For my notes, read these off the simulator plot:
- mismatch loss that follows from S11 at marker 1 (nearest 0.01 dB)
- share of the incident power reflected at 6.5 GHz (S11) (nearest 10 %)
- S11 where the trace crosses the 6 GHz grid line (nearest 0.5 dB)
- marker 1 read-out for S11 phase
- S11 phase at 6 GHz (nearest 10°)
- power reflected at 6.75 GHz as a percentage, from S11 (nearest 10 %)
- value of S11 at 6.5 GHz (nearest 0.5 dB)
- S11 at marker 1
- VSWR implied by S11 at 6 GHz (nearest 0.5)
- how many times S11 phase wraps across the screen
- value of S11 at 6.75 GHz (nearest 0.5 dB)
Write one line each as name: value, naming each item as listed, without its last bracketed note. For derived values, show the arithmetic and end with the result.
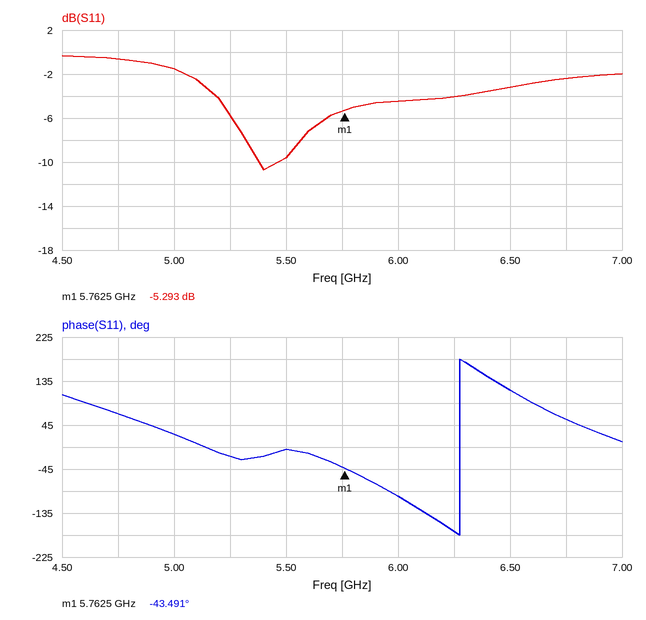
mismatch loss that follows from S11 at marker 1: −10 log10(1 − 10^(-5.293/10)) ≈ 1.52 dB
share of the incident power reflected at 6.5 GHz (S11): 10^(-3/10) ≈ 50 %
S11 where the trace crosses the 6 GHz grid line: -4.5 dB
marker 1 read-out for S11 phase: -43.491°
S11 phase at 6 GHz: -100°
power reflected at 6.75 GHz as a percentage, from S11: 10^(-2.5/10) ≈ 56.2 %, so 60 % to the nearest 10 %
value of S11 at 6.5 GHz: -3.0 dB
S11 at marker 1: -5.293 dB
VSWR implied by S11 at 6 GHz: |Γ| = 10^(-4.5/20) = 0.5957; VSWR = (1 + 0.5957)/(1 − 0.5957) ≈ 4.0
how many times S11 phase wraps across the screen: 1
value of S11 at 6.75 GHz: -2.5 dB
